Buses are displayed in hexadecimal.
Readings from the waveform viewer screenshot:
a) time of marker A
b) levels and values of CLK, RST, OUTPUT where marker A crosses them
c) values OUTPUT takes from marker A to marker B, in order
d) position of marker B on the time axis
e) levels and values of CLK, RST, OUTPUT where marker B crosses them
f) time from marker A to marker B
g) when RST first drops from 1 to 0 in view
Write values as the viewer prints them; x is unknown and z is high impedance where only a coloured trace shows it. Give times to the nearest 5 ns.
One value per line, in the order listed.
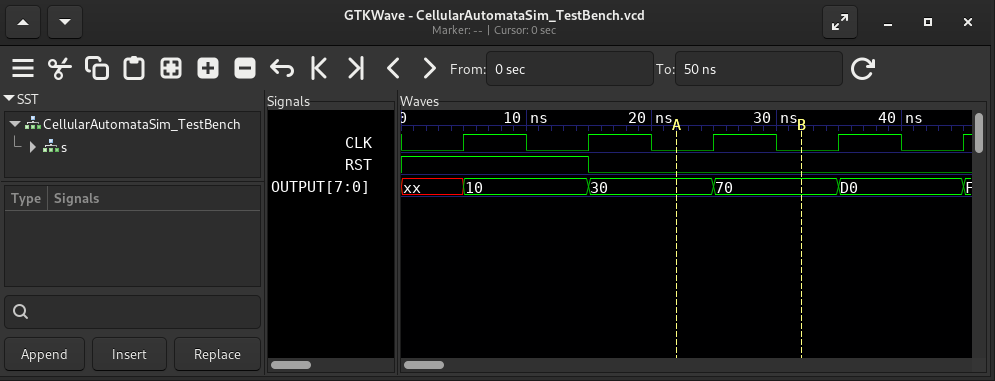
20 ns
CLK=0, RST=0, OUTPUT=30
30, 70
30 ns
CLK=0, RST=0, OUTPUT=70
10 ns
15 ns
